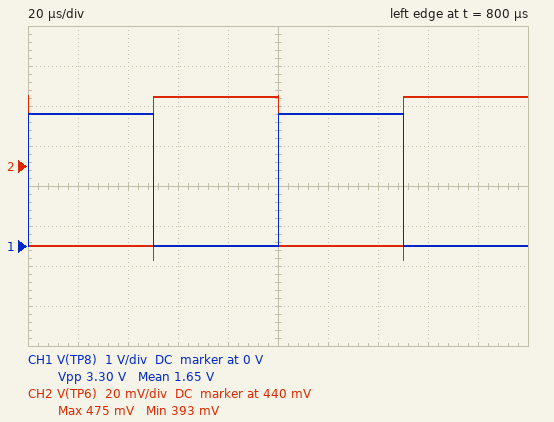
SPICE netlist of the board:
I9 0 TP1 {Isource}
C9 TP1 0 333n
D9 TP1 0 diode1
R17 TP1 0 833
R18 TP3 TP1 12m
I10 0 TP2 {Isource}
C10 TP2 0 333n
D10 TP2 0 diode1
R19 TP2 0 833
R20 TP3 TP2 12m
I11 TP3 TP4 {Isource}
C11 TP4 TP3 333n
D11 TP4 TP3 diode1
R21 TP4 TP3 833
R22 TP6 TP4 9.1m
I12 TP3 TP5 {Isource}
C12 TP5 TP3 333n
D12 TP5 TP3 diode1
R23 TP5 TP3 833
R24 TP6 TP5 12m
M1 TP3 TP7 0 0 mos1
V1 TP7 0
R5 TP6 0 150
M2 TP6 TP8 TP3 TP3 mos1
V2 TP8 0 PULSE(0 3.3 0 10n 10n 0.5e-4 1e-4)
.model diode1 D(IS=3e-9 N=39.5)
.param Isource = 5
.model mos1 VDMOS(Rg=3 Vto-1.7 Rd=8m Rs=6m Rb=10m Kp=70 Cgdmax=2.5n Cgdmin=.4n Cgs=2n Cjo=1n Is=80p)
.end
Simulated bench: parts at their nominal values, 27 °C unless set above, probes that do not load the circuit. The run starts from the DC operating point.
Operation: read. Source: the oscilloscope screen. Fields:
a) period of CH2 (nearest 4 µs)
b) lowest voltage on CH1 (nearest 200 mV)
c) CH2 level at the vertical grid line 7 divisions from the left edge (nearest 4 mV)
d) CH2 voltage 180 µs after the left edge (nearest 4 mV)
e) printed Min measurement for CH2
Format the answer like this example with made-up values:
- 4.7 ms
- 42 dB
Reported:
- 100 µs
- 0 V
- 400 mV
- 476 mV
- 393 mV
